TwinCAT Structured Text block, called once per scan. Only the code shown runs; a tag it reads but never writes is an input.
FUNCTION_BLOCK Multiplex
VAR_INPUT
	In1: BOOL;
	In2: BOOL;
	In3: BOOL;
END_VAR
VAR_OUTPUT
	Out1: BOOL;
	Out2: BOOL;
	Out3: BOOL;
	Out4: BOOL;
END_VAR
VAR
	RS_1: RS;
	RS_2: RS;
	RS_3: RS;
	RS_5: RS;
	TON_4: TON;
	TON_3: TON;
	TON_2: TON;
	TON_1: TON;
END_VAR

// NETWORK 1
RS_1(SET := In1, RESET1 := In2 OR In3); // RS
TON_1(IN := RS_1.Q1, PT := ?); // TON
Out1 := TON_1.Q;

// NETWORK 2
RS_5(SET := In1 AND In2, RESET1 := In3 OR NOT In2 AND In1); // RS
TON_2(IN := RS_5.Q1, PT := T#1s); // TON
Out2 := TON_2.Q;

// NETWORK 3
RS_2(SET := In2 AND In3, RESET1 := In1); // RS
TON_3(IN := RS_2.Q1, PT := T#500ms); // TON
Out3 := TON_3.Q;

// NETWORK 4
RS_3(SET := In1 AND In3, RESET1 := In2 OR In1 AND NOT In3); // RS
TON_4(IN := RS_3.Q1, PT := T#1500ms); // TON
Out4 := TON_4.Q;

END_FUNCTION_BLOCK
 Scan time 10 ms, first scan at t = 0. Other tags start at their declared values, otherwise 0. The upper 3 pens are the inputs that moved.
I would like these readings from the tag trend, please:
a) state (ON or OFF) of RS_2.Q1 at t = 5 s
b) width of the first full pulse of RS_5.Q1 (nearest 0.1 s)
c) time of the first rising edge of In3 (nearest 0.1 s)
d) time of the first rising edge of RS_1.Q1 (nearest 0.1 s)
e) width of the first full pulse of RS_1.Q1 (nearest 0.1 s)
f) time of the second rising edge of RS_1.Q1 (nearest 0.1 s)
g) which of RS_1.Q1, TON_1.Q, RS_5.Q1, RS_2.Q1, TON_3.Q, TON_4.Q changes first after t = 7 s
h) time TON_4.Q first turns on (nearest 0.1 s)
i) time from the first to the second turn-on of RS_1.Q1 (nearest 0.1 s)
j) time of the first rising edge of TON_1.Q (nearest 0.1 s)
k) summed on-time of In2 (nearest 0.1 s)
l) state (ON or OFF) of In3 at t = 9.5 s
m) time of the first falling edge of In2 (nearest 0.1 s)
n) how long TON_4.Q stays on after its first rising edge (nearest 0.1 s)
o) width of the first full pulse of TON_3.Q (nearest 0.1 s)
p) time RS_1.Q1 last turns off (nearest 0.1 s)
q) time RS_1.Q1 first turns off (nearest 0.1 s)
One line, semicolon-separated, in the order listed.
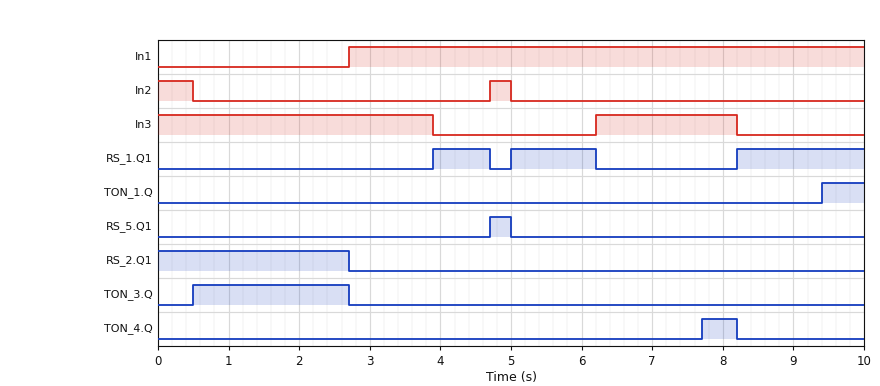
OFF; 0.3 s; 6.2 s; 3.9 s; 0.8 s; 5.0 s; TON_4.Q; 7.7 s; 1.1 s; 9.4 s; 0.8 s; OFF; 0.5 s; 0.5 s; 2.2 s; 6.2 s; 4.7 s
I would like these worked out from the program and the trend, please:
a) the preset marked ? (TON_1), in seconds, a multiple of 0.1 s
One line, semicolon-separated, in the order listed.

1.2 s
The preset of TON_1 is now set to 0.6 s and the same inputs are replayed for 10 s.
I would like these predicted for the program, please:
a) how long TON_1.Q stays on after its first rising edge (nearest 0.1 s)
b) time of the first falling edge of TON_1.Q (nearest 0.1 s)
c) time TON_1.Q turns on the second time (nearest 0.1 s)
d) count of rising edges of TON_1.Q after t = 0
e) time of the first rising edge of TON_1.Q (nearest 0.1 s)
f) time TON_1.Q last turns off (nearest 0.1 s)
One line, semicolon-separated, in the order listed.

0.2 s; 4.7 s; 5.6 s; 3; 4.5 s; 6.2 s
